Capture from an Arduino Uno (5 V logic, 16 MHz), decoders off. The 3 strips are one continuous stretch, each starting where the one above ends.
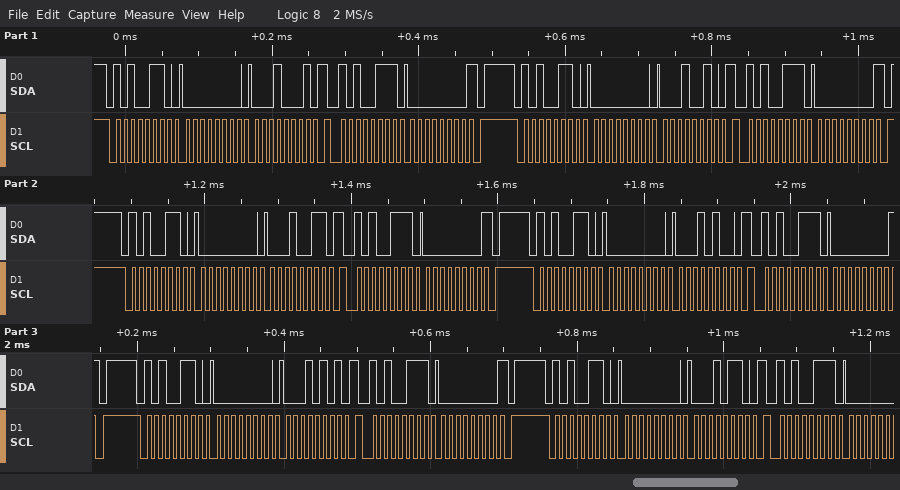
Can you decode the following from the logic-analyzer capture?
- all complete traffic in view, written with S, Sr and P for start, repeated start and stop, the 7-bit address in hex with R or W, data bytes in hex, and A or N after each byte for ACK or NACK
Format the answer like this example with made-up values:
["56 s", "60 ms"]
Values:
["S 53W A 00 A 11 A Sr 53R A 00 N P S 53W A 00 A 12 A Sr 53R A 00 N P S 53W A 00 A 13 A Sr 53R A 00 N P S 53W A 00 A 14 A Sr 53R A 00 N P S 53W A 00 A 15 A Sr 53R A 00 N P S 53W A 00 A 16 A Sr 53R A"]
